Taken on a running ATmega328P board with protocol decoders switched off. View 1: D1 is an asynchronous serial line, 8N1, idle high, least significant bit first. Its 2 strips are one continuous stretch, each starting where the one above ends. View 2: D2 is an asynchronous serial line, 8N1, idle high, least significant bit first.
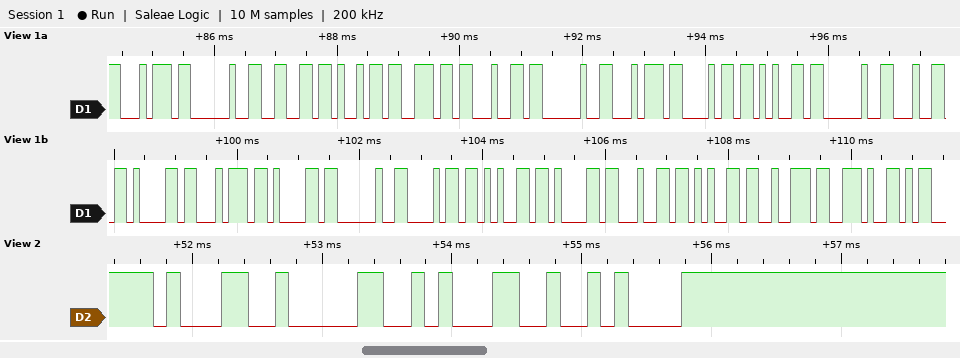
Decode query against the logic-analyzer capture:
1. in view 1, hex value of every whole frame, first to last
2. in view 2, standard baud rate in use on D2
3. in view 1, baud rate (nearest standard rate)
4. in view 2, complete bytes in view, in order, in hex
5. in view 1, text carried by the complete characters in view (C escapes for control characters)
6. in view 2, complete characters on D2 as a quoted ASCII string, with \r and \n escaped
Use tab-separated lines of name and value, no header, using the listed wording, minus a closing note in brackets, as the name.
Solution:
in view 1, hex value of every whole frame, first to last	0x74 0x20 0x66 0x69 0x6E 0x64 0x20 0x74 0x68 0x65 0x20 0x64 0x61 0x74 0x61 0x20 0x68 0x65 0x61 0x64 0x65 0x72 0x2E
in view 2, standard baud rate in use on D2	9600 baud
in view 1, baud rate	9600 baud
in view 2, complete bytes in view, in order, in hex	31 30 31 0A
in view 1, text carried by the complete characters in view	"t find the data header."
in view 2, complete characters on D2 as a quoted ASCII string, with \r and \n escaped	"101\n"
